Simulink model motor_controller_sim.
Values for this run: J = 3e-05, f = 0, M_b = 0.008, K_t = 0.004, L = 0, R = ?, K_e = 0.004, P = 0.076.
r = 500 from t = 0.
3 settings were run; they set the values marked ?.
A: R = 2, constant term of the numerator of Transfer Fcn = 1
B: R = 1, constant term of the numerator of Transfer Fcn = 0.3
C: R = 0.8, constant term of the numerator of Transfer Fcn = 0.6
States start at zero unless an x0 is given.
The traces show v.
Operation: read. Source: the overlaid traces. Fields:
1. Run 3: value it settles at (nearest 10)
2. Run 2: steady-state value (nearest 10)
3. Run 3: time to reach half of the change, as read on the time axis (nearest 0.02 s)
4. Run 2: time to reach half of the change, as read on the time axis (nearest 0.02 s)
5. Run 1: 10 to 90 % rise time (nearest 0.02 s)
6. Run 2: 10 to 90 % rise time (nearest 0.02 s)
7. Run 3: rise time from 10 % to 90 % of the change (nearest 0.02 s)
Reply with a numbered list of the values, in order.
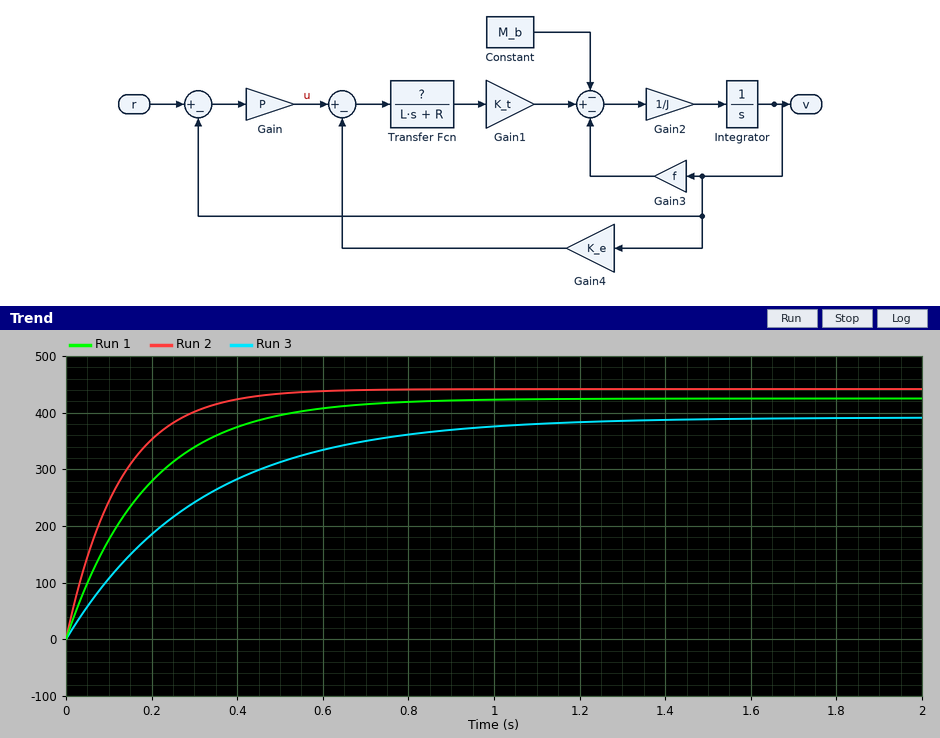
1. 390
2. 440
3. 0.22 s
4. 0.08 s
5. 0.42 s
6. 0.28 s
7. 0.68 s
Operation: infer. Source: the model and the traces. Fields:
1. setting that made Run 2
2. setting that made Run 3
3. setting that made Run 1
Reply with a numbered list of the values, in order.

1. C
2. B
3. A
